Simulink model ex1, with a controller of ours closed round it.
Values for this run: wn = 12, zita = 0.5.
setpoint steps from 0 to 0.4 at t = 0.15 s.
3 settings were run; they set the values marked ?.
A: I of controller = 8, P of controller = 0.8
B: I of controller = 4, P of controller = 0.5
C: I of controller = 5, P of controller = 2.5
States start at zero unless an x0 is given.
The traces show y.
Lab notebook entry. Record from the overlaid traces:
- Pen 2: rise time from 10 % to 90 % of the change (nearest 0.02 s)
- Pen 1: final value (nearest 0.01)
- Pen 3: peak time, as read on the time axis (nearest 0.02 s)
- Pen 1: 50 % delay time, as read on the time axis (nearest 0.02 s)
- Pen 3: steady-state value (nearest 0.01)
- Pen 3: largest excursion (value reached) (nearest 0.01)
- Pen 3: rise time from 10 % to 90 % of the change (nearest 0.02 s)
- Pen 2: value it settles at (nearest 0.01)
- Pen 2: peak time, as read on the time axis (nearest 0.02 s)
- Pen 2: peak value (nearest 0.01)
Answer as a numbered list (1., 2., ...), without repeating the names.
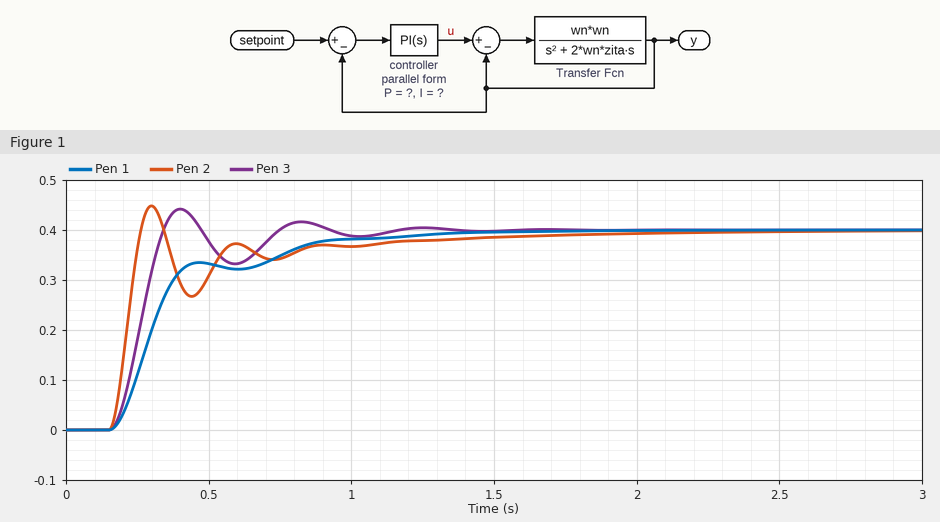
1. 0.08 s
2. 0.40
3. 0.40 s
4. 0.30 s
5. 0.40
6. 0.44
7. 0.12 s
8. 0.40
9. 0.30 s
10. 0.45
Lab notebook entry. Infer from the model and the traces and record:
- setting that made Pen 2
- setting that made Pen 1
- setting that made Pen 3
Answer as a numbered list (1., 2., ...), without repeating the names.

1. C
2. B
3. A
